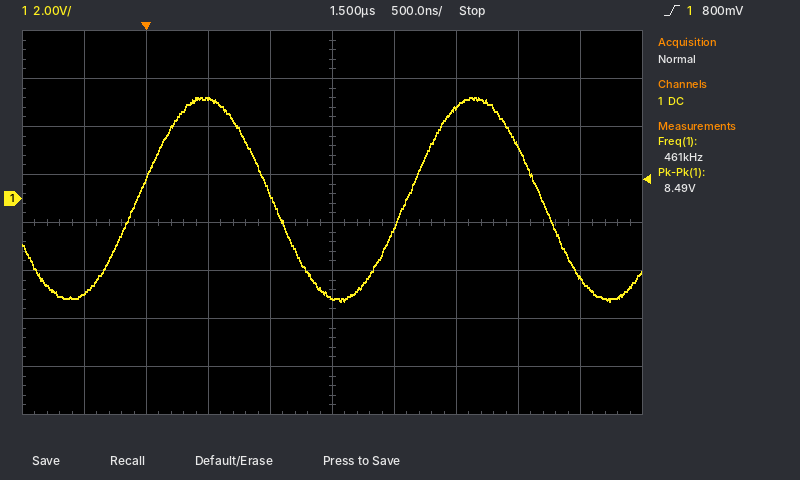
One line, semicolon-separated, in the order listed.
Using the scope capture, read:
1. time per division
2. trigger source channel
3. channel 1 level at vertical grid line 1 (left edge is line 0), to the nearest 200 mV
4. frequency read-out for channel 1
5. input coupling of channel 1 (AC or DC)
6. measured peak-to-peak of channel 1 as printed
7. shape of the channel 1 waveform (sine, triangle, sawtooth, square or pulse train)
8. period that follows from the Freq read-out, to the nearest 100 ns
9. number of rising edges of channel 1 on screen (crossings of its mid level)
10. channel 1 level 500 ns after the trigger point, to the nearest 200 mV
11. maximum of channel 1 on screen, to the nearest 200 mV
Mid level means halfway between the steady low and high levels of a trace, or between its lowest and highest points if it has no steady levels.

500 ns; channel 1; -4.0 V; 461 kHz; DC; 8.49 V; sine; 2.2 µs; 2; 4.2 V; 4.2 V
